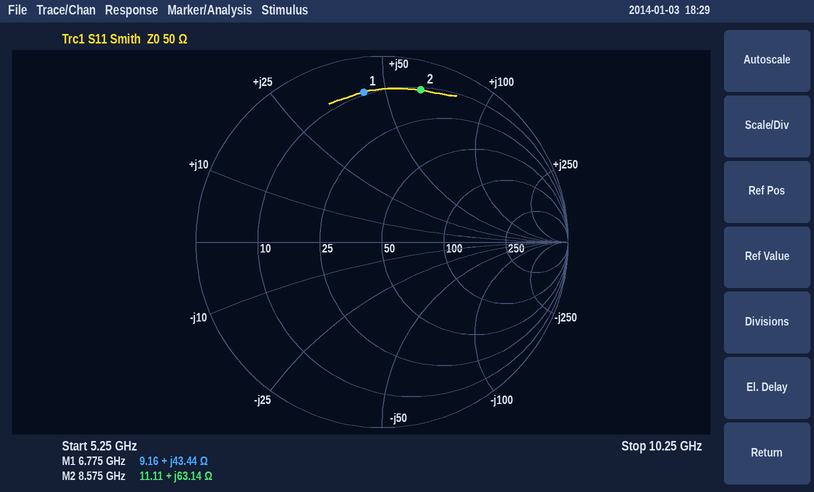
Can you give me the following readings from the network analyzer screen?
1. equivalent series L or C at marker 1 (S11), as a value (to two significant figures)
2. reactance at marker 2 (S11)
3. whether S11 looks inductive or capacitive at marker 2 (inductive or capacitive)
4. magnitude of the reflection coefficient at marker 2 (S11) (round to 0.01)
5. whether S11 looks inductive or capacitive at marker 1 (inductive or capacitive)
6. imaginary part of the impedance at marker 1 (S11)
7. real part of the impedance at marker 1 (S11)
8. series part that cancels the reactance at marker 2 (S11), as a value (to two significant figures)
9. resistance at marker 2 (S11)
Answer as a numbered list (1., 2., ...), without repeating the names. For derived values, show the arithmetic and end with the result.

1. L = 43.44 Ω/(2π × 6.775 GHz) ≈ 1.0 nH
2. +63.14 Ω
3. inductive
4. 0.84
5. inductive
6. +43.44 Ω
7. 9.16 Ω
8. C = 1/(2π × 8.575 GHz × 63.14 Ω) ≈ 294 fF, so 290 fF to two significant figures
9. 11.11 Ω
